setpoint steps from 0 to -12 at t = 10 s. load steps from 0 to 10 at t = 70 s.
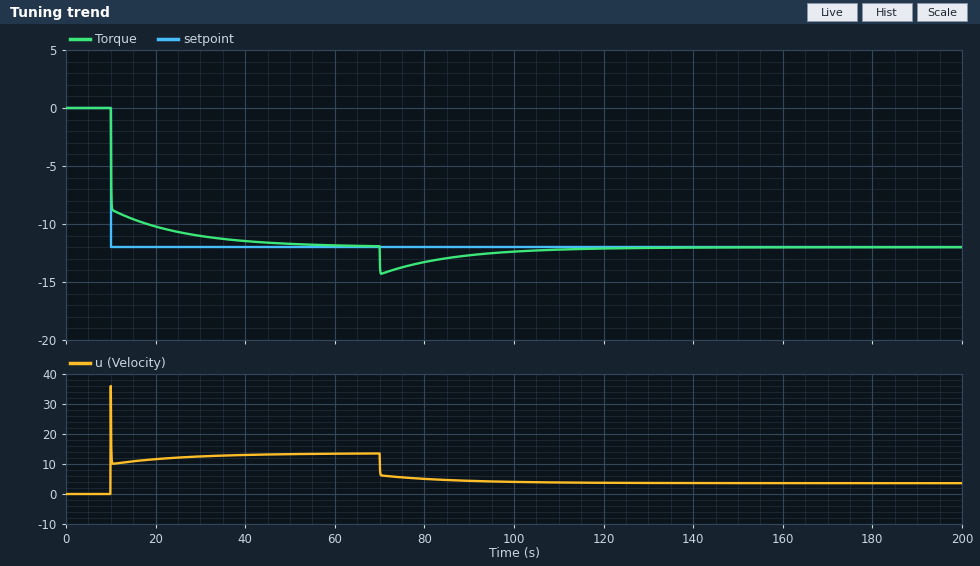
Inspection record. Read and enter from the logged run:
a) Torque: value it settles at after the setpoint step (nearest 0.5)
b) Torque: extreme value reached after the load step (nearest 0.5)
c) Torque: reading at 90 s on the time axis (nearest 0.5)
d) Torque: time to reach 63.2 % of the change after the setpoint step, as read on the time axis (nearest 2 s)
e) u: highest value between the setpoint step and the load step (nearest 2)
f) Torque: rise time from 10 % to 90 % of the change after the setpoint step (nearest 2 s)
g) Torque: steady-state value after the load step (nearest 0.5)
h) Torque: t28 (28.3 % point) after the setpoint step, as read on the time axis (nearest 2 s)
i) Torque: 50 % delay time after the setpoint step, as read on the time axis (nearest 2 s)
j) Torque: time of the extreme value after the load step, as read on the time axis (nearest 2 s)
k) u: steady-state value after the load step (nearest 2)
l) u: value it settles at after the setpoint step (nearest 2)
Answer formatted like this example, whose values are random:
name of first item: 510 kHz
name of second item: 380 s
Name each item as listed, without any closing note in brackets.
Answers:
Torque: value it settles at after the setpoint step: -12.0
Torque: extreme value reached after the load step: -14.5
Torque: reading at 90 s on the time axis: -12.5
Torque: time to reach 63.2 % of the change after the setpoint step, as read on the time axis: 10 s
u: highest value between the setpoint step and the load step: 36
Torque: rise time from 10 % to 90 % of the change after the setpoint step: 16 s
Torque: steady-state value after the load step: -12.0
Torque: t28 (28.3 % point) after the setpoint step, as read on the time axis: 10 s
Torque: 50 % delay time after the setpoint step, as read on the time axis: 10 s
Torque: time of the extreme value after the load step, as read on the time axis: 70 s
u: steady-state value after the load step: 4
u: value it settles at after the setpoint step: 14
